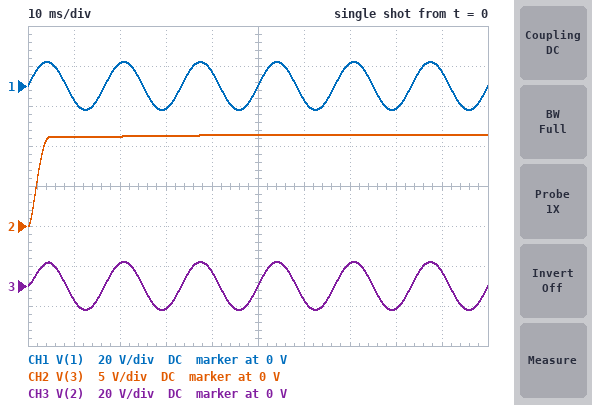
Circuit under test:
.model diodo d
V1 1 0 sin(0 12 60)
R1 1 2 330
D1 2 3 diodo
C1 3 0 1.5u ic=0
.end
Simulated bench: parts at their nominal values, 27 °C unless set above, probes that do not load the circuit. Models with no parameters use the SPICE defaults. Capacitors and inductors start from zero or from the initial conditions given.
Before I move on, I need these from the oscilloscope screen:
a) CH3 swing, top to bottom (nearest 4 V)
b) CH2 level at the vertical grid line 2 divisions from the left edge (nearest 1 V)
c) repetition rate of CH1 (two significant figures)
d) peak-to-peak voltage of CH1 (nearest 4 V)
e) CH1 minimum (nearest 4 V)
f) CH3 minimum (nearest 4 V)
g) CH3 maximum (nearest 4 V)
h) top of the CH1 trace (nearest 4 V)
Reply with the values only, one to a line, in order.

24 V
11 V
60 Hz
24 V
-12 V
-12 V
12 V
12 V
